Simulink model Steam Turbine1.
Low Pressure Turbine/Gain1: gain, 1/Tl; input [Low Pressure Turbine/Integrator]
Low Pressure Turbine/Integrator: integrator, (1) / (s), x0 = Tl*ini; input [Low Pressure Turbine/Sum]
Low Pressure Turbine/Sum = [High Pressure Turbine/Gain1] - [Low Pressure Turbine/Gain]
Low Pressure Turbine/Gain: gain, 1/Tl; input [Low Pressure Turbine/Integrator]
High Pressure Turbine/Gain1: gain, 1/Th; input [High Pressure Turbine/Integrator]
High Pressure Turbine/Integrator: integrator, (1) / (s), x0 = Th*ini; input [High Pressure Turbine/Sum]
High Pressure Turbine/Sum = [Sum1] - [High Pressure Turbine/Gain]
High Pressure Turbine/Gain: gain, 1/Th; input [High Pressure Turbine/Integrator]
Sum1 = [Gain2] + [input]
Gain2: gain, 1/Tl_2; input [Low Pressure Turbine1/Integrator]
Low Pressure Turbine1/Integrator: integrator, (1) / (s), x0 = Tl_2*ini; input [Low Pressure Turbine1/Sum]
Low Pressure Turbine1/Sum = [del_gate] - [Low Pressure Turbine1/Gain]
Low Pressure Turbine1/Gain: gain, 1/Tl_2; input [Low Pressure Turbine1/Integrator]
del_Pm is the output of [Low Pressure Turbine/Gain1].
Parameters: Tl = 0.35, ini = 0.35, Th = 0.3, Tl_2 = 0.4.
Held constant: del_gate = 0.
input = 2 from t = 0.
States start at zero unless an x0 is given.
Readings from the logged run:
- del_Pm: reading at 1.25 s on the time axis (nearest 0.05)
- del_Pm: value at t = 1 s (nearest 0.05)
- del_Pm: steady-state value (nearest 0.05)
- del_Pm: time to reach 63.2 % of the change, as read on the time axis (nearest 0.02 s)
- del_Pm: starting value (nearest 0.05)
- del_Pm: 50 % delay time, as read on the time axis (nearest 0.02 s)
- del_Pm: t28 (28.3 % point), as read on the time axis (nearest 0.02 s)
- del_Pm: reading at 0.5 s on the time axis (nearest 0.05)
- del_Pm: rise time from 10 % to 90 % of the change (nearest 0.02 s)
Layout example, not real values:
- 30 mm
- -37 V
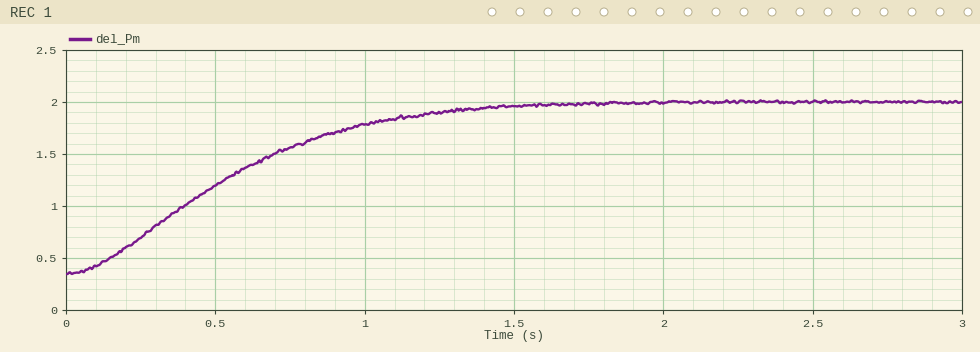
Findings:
- 1.90
- 1.80
- 2.00
- 0.62 s
- 0.35
- 0.48 s
- 0.30 s
- 1.20
- 0.94 s
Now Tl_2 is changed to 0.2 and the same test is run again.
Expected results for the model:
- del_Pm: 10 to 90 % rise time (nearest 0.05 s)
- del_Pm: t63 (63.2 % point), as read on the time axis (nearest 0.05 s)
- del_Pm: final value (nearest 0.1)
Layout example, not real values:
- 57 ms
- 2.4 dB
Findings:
- 1.05 s
- 0.65 s
- 2.0
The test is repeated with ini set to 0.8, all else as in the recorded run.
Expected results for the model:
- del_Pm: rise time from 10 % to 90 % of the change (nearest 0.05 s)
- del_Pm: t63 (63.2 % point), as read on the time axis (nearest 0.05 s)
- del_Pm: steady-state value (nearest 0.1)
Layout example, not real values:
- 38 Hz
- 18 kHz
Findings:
- 0.65 s
- 0.50 s
- 2.0
